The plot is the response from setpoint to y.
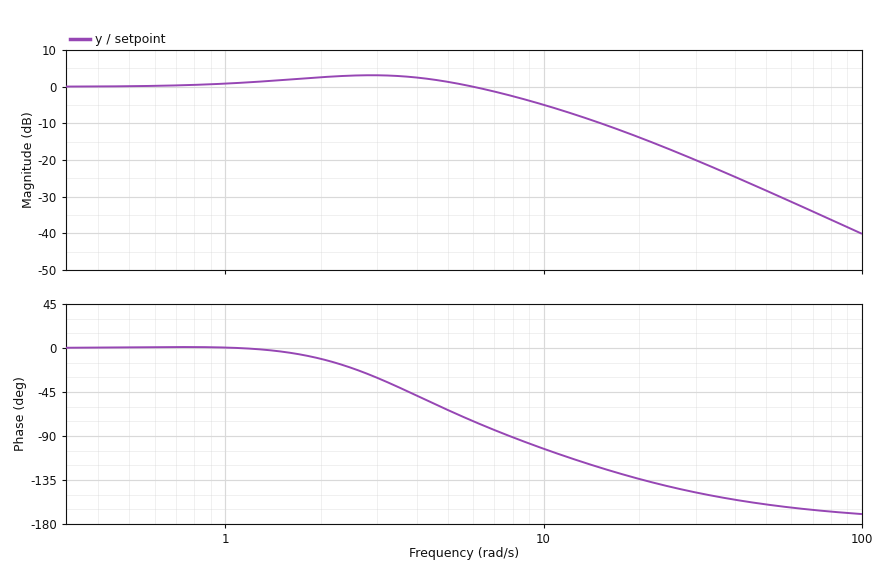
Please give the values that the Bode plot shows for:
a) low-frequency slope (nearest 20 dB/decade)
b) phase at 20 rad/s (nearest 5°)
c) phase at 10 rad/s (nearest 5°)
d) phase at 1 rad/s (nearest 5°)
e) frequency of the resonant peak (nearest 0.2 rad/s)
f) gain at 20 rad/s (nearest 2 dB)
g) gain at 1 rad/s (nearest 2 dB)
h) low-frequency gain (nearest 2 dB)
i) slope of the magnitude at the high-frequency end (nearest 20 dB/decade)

0 dB/decade
-135°
-105°
0°
2.8 rad/s
-14 dB
0 dB
0 dB
-40 dB/decade
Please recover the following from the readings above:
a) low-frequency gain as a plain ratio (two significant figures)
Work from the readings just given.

1.0
